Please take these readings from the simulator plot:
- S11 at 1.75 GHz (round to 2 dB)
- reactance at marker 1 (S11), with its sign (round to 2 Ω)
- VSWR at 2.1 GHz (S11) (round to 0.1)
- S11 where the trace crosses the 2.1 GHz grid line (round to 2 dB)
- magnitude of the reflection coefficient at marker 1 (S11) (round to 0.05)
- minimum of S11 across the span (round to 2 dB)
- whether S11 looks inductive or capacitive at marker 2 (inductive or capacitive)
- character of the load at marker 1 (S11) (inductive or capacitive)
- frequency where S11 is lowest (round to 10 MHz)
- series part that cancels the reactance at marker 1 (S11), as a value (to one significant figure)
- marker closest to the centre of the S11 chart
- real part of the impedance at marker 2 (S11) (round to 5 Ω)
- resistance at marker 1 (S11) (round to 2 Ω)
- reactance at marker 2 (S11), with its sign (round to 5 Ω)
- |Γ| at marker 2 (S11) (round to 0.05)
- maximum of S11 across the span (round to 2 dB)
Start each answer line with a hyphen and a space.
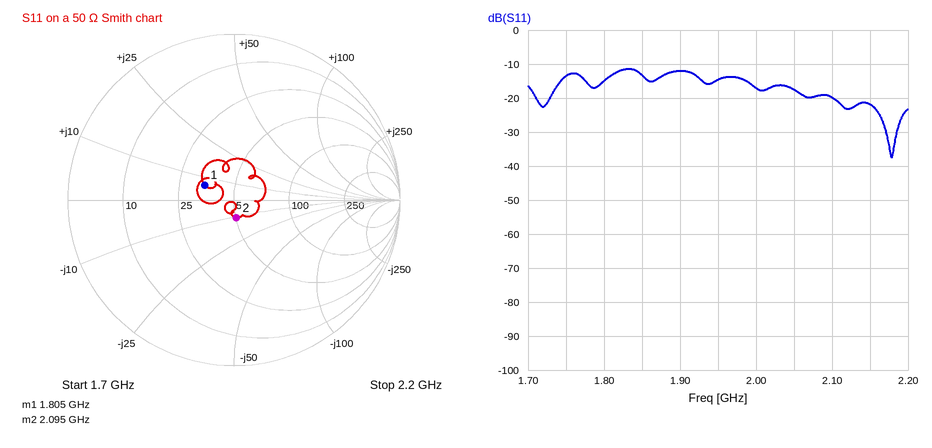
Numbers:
- -14 dB
- +6 Ω
- 1.2
- -20 dB
- 0.20
- -38 dB
- capacitive
- inductive
- 2.18 GHz
- 10 pF
- marker 2
- 50 Ω
- 34 Ω
- -10 Ω
- 0.10
- -12 dB
